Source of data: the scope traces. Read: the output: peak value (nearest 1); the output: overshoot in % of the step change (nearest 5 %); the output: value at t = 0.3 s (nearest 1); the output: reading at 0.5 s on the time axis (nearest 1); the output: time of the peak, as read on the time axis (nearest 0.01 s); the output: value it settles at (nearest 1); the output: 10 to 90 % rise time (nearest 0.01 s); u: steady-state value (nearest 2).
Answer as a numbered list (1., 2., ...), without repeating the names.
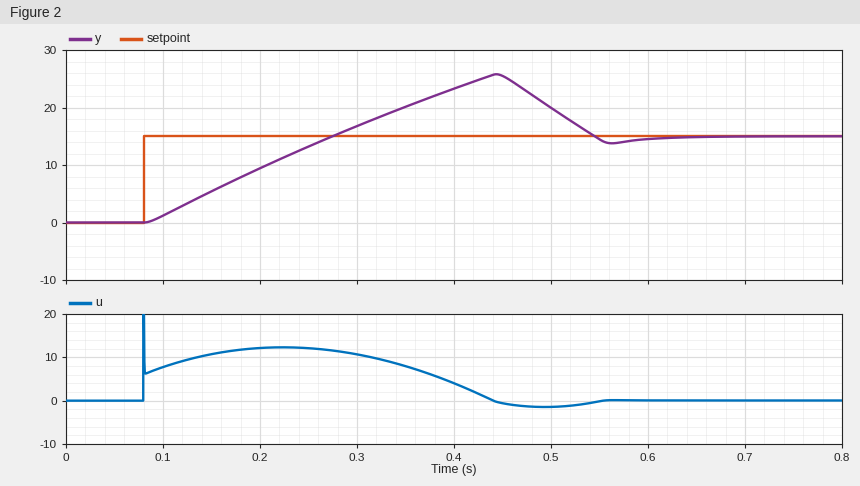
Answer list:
1. 26
2. 70 %
3. 17
4. 20
5. 0.44 s
6. 15
7. 0.15 s
8. 0
